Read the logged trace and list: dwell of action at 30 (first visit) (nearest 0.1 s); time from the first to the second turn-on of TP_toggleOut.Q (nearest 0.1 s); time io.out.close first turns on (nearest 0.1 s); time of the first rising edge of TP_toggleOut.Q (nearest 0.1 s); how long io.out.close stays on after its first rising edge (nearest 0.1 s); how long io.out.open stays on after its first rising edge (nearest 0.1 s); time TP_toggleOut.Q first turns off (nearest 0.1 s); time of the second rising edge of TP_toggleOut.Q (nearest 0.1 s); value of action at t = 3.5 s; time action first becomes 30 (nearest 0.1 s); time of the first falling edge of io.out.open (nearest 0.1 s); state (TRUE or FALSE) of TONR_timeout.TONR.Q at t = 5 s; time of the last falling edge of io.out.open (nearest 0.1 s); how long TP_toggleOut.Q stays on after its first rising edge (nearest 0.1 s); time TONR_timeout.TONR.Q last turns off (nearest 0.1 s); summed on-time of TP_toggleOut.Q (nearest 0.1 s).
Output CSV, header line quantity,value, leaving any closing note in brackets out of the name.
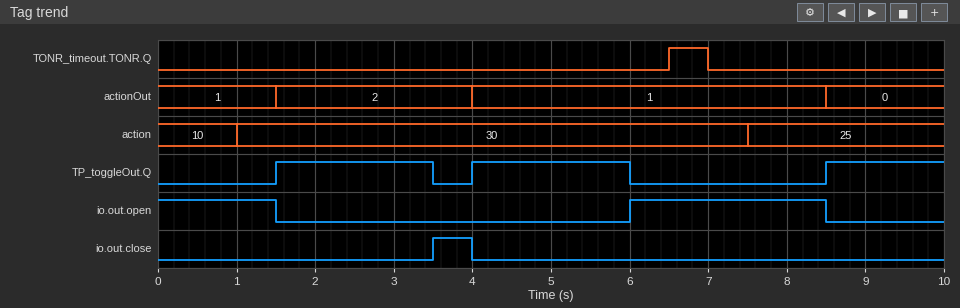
quantity,value
dwell of action at 30 (first visit),6.5 s
time from the first to the second turn-on of TP_toggleOut.Q,2.5 s
time io.out.close first turns on,3.5 s
time of the first rising edge of TP_toggleOut.Q,1.5 s
how long io.out.close stays on after its first rising edge,0.5 s
how long io.out.open stays on after its first rising edge,2.5 s
time TP_toggleOut.Q first turns off,3.5 s
time of the second rising edge of TP_toggleOut.Q,4.0 s
value of action at t = 3.5 s,30
time action first becomes 30,1.0 s
time of the first falling edge of io.out.open,1.5 s
state (TRUE or FALSE) of TONR_timeout.TONR.Q at t = 5 s,FALSE
time of the last falling edge of io.out.open,8.5 s
how long TP_toggleOut.Q stays on after its first rising edge,2.0 s
time TONR_timeout.TONR.Q last turns off,7.0 s
summed on-time of TP_toggleOut.Q,5.5 s
